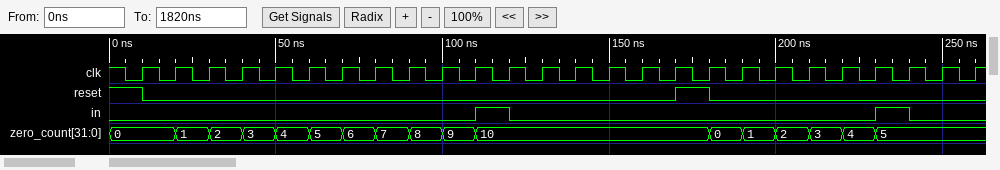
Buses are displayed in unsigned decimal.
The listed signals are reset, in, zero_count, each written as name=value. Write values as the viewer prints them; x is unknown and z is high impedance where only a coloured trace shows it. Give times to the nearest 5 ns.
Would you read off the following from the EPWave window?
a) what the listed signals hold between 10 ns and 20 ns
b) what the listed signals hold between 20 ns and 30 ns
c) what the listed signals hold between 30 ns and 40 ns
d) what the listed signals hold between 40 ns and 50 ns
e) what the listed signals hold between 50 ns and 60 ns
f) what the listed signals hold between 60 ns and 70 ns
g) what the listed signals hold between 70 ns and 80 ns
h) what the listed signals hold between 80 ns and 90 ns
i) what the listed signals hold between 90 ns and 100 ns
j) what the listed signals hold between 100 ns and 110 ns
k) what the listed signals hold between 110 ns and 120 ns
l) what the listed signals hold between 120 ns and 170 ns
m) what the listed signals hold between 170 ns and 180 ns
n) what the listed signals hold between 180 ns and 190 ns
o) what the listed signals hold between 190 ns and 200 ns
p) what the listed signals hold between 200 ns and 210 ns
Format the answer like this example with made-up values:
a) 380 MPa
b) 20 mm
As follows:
a) reset=0, in=0, zero_count=0
b) reset=0, in=0, zero_count=1
c) reset=0, in=0, zero_count=2
d) reset=0, in=0, zero_count=3
e) reset=0, in=0, zero_count=4
f) reset=0, in=0, zero_count=5
g) reset=0, in=0, zero_count=6
h) reset=0, in=0, zero_count=7
i) reset=0, in=0, zero_count=8
j) reset=0, in=0, zero_count=9
k) reset=0, in=1, zero_count=10
l) reset=0, in=0, zero_count=10
m) reset=1, in=0, zero_count=10
n) reset=0, in=0, zero_count=0
o) reset=0, in=0, zero_count=1
p) reset=0, in=0, zero_count=2
